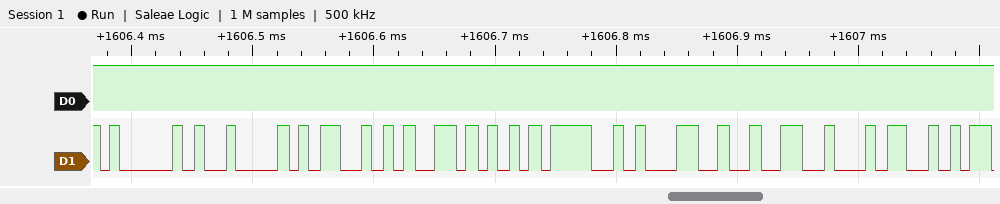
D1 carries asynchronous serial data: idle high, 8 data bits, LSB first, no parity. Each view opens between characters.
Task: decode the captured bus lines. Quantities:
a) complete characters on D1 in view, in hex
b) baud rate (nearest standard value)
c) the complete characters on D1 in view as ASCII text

41, 42, 53, 56, 3D, 31, 32, 34
115200 baud
"ABSV=124"
